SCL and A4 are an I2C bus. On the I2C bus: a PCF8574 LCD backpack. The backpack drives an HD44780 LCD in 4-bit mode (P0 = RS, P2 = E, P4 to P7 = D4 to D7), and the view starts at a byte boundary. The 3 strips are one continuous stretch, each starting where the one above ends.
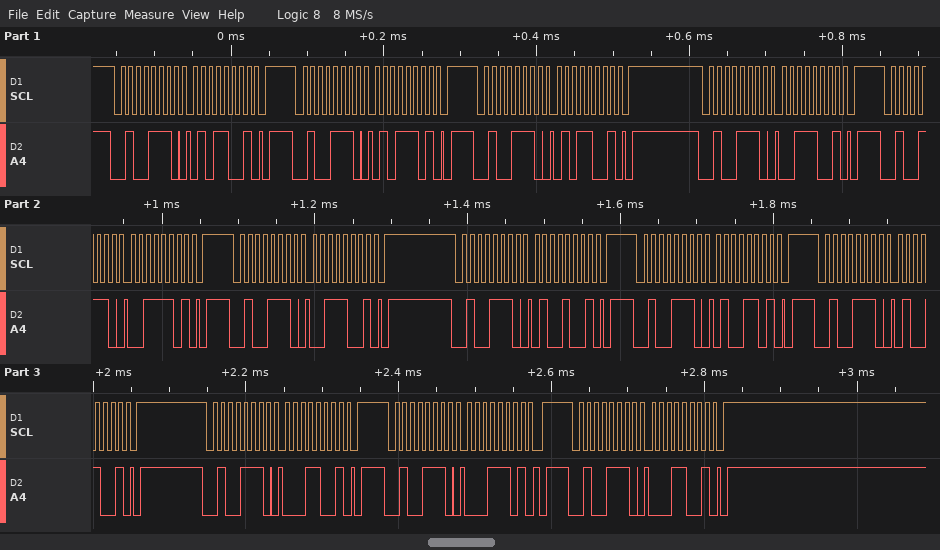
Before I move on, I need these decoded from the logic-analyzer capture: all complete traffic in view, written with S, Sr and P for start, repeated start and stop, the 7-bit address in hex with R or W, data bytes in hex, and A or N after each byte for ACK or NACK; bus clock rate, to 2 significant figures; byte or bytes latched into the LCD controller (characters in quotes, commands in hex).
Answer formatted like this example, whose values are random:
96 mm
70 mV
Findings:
S 27W A 59 A P S 27W A 5D A P S 27W A 59 A P S 27W A 39 A P S 27W A 3D A P S 27W A 39 A P S 27W A 49 A P S 27W A 4D A P S 27W A 49 A P S 27W A 19 A P S 27W A 1D A P S 27W A 19 A P
100 kHz
'S' 'A'
